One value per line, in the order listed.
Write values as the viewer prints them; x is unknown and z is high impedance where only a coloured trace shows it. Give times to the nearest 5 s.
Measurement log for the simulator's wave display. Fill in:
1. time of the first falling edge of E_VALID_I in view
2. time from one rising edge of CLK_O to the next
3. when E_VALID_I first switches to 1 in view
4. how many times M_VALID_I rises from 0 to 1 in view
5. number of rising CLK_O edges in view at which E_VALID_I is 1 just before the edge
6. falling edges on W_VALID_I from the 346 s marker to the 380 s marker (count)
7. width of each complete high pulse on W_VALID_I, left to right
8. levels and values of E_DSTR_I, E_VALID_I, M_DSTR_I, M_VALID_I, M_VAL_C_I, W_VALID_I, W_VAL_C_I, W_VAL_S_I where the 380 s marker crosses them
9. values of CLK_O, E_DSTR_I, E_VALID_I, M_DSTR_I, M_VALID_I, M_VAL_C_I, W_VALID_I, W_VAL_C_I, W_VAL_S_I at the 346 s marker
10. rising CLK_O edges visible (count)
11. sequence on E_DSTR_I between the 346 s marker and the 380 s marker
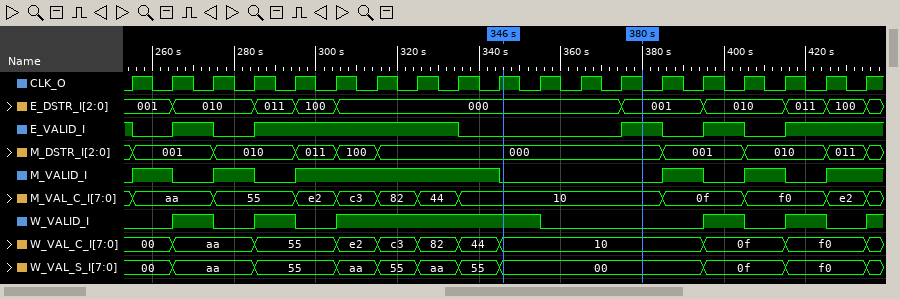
255 s
10 s
265 s
6
11
1
10 s, 10 s, 50 s, 10 s, 10 s
E_DSTR_I=001, E_VALID_I=1, M_DSTR_I=000, M_VALID_I=0, M_VAL_C_I=10, W_VALID_I=0, W_VAL_C_I=10, W_VAL_S_I=00
CLK_O=1, E_DSTR_I=000, E_VALID_I=0, M_DSTR_I=000, M_VALID_I=0, M_VAL_C_I=10, W_VALID_I=1, W_VAL_C_I=10, W_VAL_S_I=00
19
000, 001
